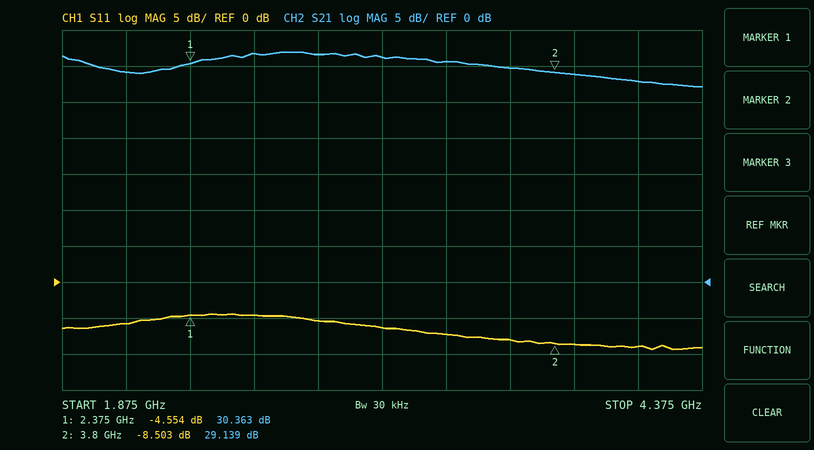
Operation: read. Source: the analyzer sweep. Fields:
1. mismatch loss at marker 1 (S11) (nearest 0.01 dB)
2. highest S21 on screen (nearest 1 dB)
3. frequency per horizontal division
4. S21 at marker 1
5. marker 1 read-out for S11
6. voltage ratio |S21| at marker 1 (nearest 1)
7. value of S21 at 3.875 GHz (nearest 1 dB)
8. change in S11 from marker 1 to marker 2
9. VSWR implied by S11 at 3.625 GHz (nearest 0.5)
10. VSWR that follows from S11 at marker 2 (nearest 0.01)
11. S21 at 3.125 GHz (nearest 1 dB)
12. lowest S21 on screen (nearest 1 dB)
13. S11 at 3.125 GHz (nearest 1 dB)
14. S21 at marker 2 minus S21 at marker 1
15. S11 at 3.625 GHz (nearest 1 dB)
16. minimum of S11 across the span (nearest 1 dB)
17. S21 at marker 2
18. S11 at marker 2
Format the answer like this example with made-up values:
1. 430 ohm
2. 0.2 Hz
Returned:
1. 1.87 dB
2. 32 dB
3. 250 MHz
4. 30.363 dB
5. -4.554 dB
6. 33
7. 29 dB
8. -3.949 dB
9. 2.5
10. 2.20
11. 31 dB
12. 27 dB
13. -6 dB
14. -1.224 dB
15. -8 dB
16. -9 dB
17. 29.139 dB
18. -8.503 dB
